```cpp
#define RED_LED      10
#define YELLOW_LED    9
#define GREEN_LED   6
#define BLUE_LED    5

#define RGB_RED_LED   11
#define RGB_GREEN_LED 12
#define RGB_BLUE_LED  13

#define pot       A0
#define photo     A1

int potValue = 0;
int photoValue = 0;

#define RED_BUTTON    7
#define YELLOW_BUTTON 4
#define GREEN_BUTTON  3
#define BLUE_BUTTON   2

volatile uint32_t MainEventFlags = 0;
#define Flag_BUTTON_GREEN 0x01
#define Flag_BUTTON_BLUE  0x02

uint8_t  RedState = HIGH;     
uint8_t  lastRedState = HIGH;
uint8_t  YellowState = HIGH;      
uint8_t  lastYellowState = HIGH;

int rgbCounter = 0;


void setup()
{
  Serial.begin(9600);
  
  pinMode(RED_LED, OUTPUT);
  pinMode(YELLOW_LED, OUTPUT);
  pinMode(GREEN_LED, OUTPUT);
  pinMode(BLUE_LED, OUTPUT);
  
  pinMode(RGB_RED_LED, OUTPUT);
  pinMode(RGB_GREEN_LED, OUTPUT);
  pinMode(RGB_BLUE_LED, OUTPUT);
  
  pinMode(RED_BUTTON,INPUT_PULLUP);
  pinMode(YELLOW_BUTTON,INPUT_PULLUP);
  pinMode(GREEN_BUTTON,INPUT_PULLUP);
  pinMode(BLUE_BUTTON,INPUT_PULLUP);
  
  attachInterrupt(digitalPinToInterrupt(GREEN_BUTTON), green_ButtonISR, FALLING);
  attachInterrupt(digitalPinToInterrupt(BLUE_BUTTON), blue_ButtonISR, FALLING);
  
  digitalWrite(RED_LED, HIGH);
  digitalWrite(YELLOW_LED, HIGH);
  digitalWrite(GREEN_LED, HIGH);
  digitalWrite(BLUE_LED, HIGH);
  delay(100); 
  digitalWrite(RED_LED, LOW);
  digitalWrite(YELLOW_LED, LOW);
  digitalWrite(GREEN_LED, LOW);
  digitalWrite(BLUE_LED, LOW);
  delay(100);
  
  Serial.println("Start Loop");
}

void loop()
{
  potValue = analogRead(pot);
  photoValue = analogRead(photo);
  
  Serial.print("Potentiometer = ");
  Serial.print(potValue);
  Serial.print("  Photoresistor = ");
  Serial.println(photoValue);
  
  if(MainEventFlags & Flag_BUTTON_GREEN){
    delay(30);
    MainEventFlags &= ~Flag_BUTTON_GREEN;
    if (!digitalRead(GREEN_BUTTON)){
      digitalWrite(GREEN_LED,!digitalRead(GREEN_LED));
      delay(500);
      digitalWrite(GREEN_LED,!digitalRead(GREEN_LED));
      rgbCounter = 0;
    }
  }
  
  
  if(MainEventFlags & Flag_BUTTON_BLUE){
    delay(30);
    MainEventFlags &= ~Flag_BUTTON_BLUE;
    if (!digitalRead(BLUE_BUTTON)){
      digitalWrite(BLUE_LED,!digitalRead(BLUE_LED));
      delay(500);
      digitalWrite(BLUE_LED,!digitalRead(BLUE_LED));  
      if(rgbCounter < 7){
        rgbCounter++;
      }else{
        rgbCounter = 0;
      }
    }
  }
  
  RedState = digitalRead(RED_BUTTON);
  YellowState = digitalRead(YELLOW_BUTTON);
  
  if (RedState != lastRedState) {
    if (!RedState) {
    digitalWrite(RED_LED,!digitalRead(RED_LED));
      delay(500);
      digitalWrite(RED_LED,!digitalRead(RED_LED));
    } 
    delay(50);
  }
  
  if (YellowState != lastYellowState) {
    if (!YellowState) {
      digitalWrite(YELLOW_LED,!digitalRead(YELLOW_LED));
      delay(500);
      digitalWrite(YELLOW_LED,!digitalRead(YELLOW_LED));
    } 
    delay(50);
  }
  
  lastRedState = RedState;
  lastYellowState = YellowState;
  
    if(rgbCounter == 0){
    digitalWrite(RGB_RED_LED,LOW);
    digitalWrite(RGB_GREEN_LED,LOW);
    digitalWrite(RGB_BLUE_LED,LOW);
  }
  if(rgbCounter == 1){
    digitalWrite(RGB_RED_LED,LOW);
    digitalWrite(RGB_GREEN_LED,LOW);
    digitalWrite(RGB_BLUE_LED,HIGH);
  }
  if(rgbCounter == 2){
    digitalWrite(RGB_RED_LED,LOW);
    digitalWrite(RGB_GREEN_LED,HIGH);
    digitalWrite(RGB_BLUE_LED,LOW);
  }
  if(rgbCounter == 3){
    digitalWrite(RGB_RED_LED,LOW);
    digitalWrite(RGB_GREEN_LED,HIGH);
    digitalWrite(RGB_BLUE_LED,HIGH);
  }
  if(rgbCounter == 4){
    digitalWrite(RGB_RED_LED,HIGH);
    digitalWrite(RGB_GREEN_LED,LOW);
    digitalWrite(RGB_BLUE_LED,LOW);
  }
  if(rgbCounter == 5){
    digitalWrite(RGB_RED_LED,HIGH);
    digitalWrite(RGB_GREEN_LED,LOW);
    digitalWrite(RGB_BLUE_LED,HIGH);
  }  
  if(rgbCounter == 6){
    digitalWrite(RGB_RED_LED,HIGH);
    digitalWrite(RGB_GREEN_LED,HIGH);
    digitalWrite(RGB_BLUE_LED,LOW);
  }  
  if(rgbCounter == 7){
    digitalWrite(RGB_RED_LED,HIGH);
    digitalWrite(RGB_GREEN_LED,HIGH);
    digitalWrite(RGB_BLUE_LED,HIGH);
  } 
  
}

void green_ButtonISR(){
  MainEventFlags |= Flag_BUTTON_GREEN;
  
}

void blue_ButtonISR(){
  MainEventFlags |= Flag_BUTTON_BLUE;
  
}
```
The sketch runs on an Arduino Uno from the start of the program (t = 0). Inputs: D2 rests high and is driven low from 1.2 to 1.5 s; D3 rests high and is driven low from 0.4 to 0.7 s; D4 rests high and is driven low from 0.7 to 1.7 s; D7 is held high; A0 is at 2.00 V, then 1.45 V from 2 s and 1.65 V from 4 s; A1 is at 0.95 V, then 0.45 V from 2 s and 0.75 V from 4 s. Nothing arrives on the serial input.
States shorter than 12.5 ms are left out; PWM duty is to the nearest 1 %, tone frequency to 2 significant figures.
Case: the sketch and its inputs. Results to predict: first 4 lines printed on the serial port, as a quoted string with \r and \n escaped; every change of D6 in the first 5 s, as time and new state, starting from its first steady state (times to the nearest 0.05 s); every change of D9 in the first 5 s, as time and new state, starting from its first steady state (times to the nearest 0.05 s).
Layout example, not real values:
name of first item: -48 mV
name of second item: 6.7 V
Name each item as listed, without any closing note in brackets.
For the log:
first 4 lines printed on the serial port, as a quoted string with \r and \n escaped: "Start Loop\r\nPotentiometer = 409  Photoresistor = 194\r\nPotentiometer = 409  Photoresistor = 194\r\nPotentiometer = 409  Photoresistor = 194\r\n"
every change of D6 in the first 5 s, as time and new state, starting from its first steady state: 0 s high; 0.1 s low; 0.45 s high; 0.95 s low
every change of D9 in the first 5 s, as time and new state, starting from its first steady state: 0 s high; 0.1 s low; 0.95 s high; 1.45 s low
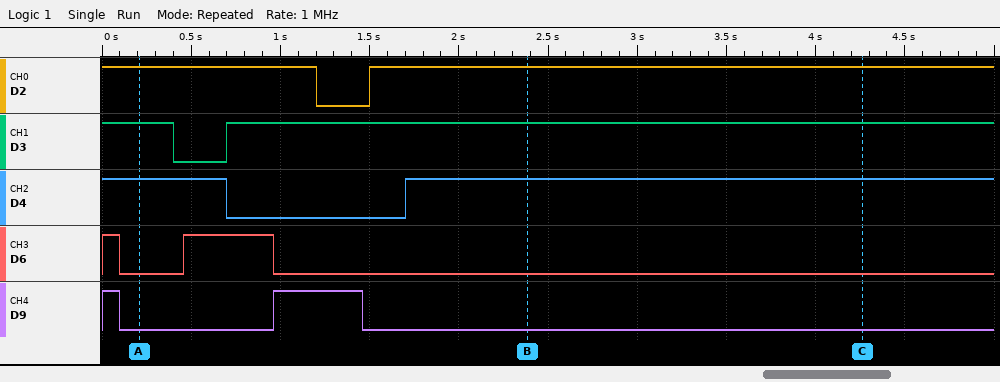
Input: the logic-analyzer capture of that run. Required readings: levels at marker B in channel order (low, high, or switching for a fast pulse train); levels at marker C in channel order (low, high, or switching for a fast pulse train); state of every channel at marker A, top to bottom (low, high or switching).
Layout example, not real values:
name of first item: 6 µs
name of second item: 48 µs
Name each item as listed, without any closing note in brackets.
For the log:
levels at marker B in channel order: D2 high, D3 high, D4 high, D6 low, D9 low
levels at marker C in channel order: D2 high, D3 high, D4 high, D6 low, D9 low
state of every channel at marker A, top to bottom: D2 high, D3 high, D4 high, D6 low, D9 low
